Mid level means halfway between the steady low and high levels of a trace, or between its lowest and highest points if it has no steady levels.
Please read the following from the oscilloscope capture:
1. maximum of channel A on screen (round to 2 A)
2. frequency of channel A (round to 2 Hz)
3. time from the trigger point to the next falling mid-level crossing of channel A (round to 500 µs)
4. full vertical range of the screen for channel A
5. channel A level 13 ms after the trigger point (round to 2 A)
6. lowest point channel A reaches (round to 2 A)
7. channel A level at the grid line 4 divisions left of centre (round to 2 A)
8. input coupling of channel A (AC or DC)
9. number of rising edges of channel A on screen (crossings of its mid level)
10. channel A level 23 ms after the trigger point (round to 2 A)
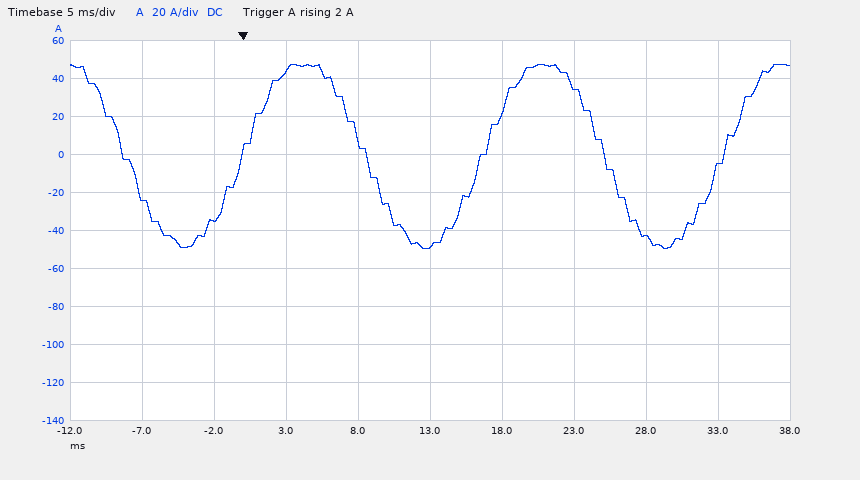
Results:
48 A
60 Hz
8.5 ms
200 A
-48 A
-50 A
-22 A
DC
3
36 A
